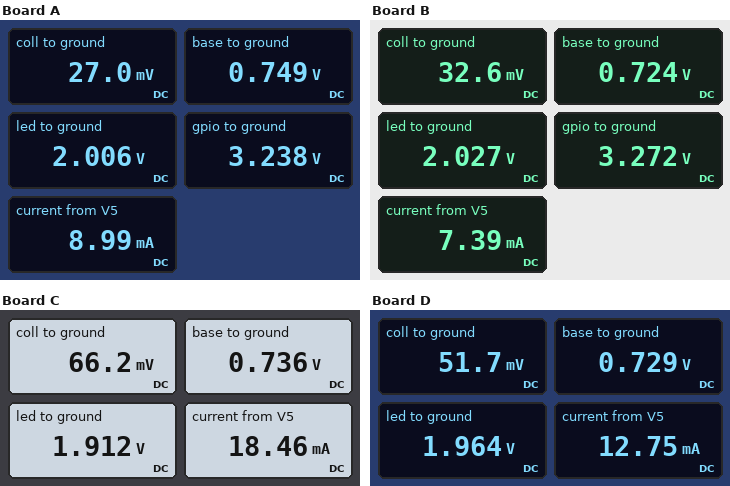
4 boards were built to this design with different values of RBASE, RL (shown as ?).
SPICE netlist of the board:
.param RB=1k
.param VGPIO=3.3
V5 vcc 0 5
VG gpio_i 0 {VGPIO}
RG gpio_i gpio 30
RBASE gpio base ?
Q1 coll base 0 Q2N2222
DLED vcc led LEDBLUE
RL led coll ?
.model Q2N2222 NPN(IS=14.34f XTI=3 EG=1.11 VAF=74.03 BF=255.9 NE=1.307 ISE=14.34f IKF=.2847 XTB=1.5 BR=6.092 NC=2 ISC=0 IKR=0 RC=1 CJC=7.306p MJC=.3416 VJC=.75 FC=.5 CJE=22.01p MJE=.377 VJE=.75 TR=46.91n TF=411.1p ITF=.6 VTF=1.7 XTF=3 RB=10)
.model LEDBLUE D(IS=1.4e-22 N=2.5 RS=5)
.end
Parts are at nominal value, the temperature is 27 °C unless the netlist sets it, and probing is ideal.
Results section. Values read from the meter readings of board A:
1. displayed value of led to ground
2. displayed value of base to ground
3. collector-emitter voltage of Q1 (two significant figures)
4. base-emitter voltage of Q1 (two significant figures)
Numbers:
2.006 V
0.749 V
27 mV
750 mV
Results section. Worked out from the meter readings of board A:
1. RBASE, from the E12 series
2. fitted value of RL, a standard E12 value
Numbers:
1.2 kΩ
220 Ω
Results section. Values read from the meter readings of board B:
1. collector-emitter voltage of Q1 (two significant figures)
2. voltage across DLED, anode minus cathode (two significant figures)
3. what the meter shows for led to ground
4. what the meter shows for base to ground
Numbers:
33 mV
3.0 V
2.027 V
0.724 V
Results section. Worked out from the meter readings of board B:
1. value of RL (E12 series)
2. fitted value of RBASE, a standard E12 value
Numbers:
270 Ω
2.7 kΩ
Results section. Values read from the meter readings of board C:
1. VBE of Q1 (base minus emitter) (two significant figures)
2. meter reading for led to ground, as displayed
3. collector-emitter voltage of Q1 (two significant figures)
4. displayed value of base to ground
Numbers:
740 mV
1.912 V
66 mV
0.736 V
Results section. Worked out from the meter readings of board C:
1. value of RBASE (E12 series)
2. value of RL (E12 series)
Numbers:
3.3 kΩ
100 Ω
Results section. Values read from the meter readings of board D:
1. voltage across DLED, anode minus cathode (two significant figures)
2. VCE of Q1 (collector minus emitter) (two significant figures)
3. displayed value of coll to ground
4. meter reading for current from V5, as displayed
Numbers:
3.0 V
52 mV
51.7 mV
12.75 mA
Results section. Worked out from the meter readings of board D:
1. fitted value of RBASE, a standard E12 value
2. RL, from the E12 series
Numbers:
3.3 kΩ
150 Ω
